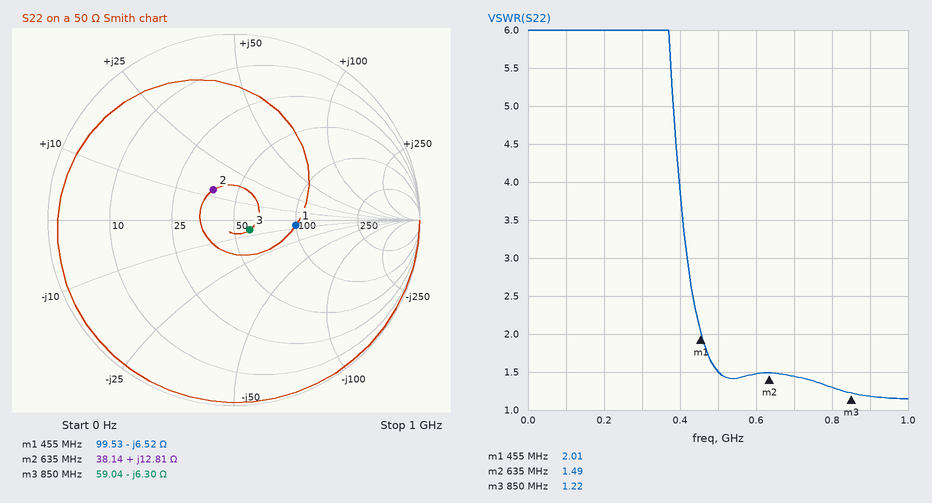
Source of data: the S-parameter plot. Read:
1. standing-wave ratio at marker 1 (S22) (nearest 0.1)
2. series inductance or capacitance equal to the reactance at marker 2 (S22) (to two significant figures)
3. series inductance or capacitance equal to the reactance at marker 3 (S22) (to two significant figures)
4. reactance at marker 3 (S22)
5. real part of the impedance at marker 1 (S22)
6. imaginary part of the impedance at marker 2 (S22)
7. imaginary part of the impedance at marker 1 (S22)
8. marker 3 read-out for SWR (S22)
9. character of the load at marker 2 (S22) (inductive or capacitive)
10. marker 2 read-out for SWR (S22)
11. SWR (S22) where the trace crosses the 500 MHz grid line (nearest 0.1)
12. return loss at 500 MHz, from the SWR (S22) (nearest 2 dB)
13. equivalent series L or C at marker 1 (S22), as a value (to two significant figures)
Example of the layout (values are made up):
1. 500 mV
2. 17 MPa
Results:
1. 2.0
2. 3.2 nH
3. 30 pF
4. -6.30 Ω
5. 99.53 Ω
6. +12.81 Ω
7. -6.52 Ω
8. 1.22
9. inductive
10. 1.49
11. 1.5
12. 14 dB
13. 54 pF
